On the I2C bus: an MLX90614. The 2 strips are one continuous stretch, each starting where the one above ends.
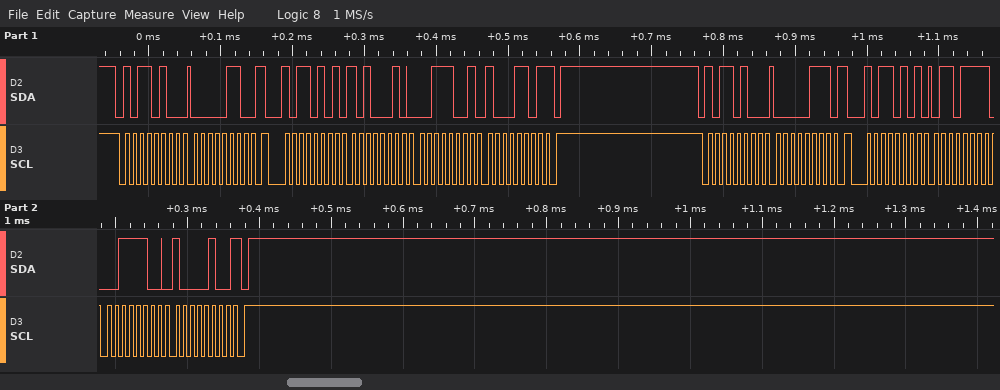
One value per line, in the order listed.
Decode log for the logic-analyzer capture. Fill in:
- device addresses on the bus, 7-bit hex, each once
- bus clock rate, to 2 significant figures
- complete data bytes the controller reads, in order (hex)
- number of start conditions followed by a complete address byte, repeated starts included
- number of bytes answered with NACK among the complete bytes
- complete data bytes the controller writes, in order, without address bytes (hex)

0x5A
100 kHz
A2 39 8D 6F 3C 84
4
2
06 07
